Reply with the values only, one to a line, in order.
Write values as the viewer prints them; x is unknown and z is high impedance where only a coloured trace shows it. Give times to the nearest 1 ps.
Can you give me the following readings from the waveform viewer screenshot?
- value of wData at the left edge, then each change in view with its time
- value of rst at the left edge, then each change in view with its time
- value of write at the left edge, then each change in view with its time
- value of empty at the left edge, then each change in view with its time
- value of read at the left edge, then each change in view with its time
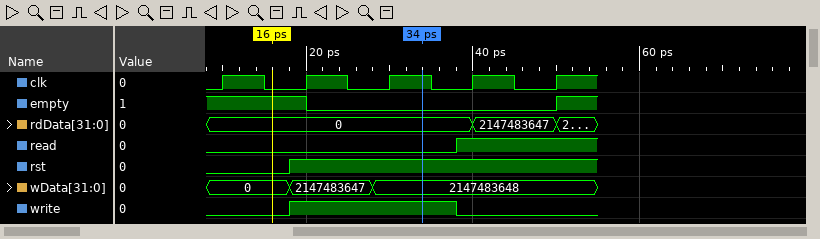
0, 2147483647 at 18 ps, 2147483648 at 28 ps
0, 1 at 18 ps
0, 1 at 18 ps, 0 at 38 ps
1, 0 at 20 ps, 1 at 50 ps
0, 1 at 38 ps
